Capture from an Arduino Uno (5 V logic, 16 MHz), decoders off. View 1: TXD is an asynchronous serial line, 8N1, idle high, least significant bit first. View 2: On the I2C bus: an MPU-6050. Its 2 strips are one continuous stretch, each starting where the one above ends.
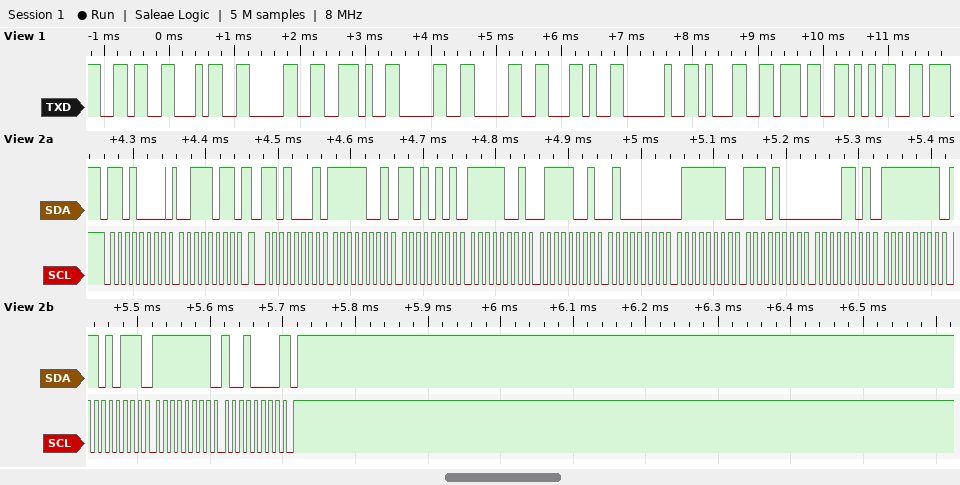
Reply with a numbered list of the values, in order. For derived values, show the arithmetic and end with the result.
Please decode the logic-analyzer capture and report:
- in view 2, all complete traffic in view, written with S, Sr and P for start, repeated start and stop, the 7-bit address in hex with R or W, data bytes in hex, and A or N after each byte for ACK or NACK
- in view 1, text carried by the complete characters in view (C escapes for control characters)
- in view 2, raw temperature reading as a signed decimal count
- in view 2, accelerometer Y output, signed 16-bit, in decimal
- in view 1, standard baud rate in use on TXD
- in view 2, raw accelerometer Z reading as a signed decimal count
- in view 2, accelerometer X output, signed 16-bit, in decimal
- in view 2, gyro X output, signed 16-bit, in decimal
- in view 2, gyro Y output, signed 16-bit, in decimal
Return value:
1. S 68W A 3B A Sr 68R A F9 A D5 A F9 A 79 A 40 A 7E A E8 A 0D A FF A D7 A FF A 90 N P
2. "640.00, 175"
3. 0xE80D = -6131
4. 0xF979 = -1671
5. 9600 baud
6. 0x407E = 16510
7. 0xF9D5 = -1579
8. 0xFFD7 = -41
9. 0xFF90 = -112
